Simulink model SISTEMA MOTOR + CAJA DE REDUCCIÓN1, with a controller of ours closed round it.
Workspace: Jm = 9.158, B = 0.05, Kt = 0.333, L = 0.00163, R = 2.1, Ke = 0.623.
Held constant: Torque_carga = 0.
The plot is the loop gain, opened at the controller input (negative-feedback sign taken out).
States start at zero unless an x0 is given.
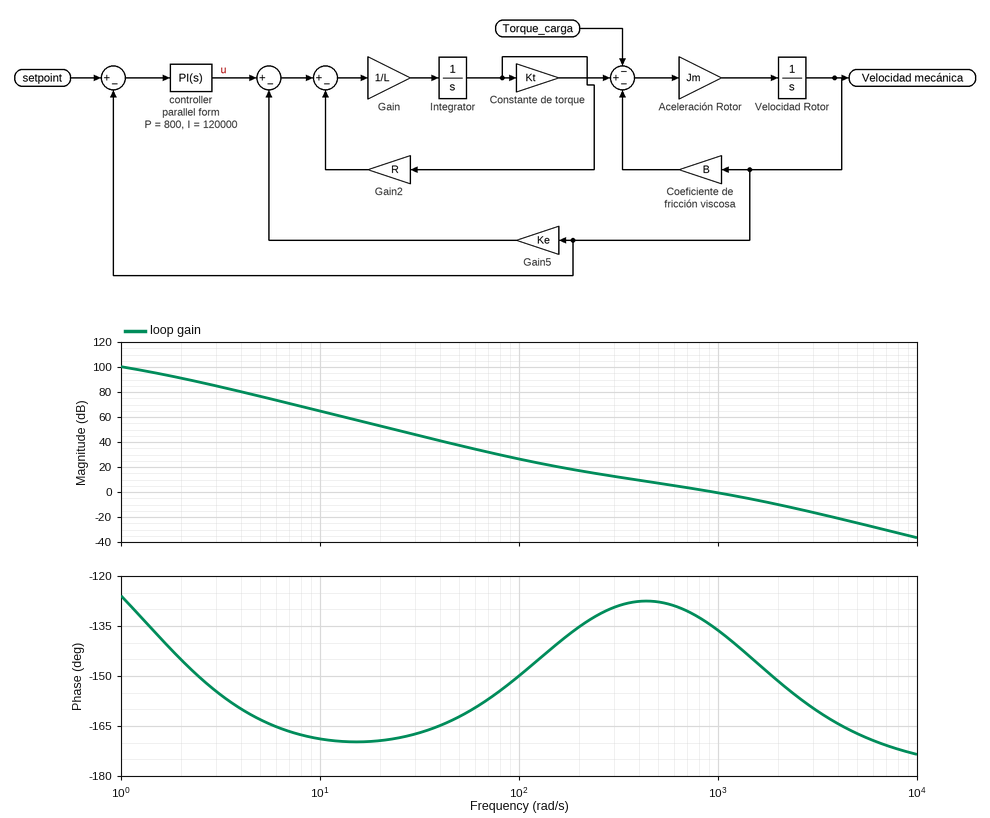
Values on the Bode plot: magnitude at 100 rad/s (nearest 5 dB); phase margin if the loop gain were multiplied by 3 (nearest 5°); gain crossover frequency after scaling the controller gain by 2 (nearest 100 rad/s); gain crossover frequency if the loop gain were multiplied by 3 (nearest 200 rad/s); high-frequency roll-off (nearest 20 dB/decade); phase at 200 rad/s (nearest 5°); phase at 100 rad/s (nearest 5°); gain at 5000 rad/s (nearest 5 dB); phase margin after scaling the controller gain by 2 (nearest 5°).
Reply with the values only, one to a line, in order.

25 dB
30°
1500 rad/s
2000 rad/s
-40 dB/decade
-135°
-150°
-25 dB
35°
